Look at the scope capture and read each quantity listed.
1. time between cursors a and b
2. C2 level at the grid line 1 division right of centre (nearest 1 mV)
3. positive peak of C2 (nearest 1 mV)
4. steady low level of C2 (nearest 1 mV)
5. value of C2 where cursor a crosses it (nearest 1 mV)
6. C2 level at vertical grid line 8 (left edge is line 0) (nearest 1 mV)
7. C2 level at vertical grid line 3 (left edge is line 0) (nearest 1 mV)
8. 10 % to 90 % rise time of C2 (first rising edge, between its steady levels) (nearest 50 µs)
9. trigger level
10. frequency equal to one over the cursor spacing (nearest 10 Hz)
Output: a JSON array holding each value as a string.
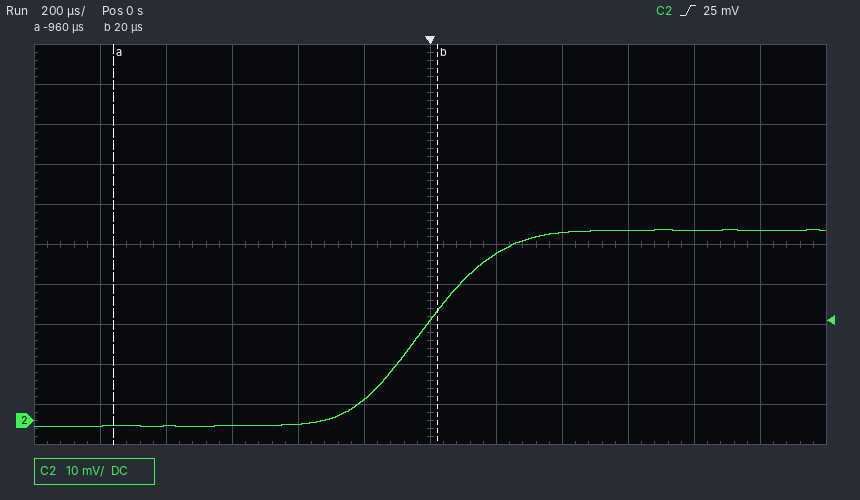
["980 µs", "42 mV", "48 mV", "-1 mV", "-1 mV", "47 mV", "-1 mV", "450 µs", "25 mV", "1.02 kHz"]
